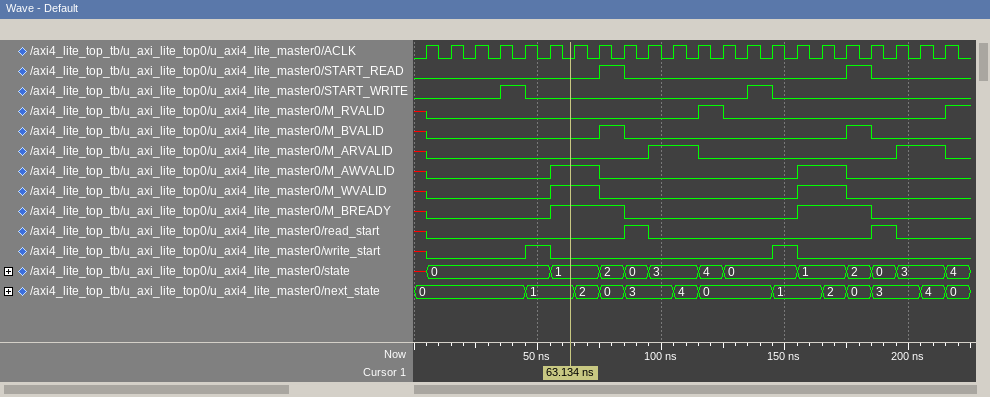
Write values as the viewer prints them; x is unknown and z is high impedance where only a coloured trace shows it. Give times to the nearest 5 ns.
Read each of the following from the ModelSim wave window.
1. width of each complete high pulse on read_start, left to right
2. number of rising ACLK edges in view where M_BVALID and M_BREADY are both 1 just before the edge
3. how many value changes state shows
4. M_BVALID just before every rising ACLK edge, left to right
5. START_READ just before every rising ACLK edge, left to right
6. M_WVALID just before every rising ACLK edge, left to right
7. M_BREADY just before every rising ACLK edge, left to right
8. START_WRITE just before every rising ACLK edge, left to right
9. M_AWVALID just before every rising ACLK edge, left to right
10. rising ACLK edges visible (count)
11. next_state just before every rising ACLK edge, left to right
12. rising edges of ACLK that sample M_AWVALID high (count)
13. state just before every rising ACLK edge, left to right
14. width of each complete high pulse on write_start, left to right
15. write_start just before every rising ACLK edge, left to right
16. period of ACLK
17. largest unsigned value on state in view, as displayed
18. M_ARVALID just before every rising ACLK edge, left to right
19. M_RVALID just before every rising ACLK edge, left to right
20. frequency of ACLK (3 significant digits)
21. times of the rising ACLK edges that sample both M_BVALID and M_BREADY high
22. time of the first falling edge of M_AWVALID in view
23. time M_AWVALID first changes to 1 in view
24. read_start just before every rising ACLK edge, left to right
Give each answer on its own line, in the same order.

10 ns, 10 ns
2
12
x 0 0 0 0 0 0 0 1 0 0 0 0 0 0 0 0 0 1 0 0 0
0 0 0 0 0 0 0 0 1 0 0 0 0 0 0 0 0 0 1 0 0 0
x 0 0 0 0 0 1 1 0 0 0 0 0 0 0 0 1 1 0 0 0 0
x 0 0 0 0 0 1 1 1 0 0 0 0 0 0 0 1 1 1 0 0 0
0 0 0 0 1 0 0 0 0 0 0 0 0 0 1 0 0 0 0 0 0 0
x 0 0 0 0 0 1 1 0 0 0 0 0 0 0 0 1 1 0 0 0 0
22
0, 0, 0, 0, 0, 1, 1, 2, 0, 3, 3, 4, 0, 0, 0, 1, 1, 2, 0, 3, 3, 4
4
x, 0, 0, 0, 0, 0, 1, 1, 2, 0, 3, 3, 4, 0, 0, 0, 1, 1, 2, 0, 3, 3
10 ns, 10 ns
x 0 0 0 0 1 0 0 0 0 0 0 0 0 0 1 0 0 0 0 0 0
10 ns
4
x 0 0 0 0 0 0 0 0 0 1 1 0 0 0 0 0 0 0 0 1 1
x 0 0 0 0 0 0 0 0 0 0 0 1 0 0 0 0 0 0 0 0 0
100 MHz
85 ns, 185 ns
75 ns
55 ns
x 0 0 0 0 0 0 0 0 1 0 0 0 0 0 0 0 0 0 1 0 0
